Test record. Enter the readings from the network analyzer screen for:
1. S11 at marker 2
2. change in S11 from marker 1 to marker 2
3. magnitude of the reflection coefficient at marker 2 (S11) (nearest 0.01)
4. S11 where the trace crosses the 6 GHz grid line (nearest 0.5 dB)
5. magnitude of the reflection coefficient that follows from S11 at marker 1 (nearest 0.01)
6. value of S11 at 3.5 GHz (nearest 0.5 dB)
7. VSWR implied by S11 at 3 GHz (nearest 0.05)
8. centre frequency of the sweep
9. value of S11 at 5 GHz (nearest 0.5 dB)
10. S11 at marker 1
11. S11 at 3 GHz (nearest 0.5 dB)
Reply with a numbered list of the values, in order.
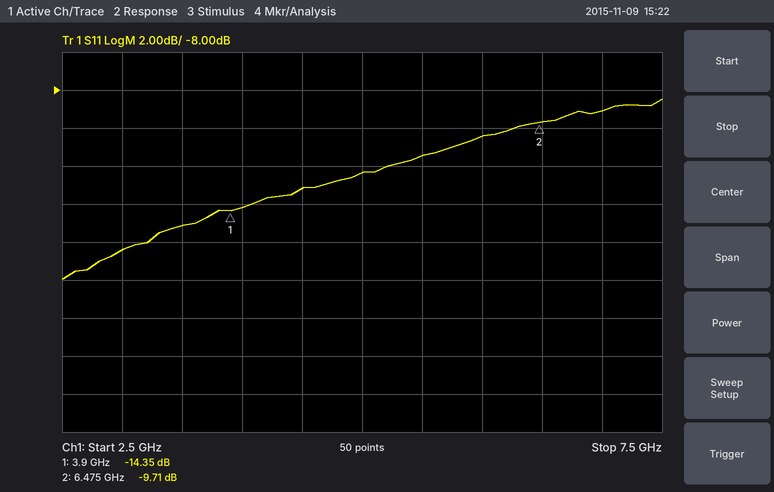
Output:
1. -9.71 dB
2. 4.64 dB
3. 0.33
4. -10.5 dB
5. 0.19
6. -15.0 dB
7. 1.35
8. 5 GHz
9. -12.5 dB
10. -14.35 dB
11. -16.5 dB
